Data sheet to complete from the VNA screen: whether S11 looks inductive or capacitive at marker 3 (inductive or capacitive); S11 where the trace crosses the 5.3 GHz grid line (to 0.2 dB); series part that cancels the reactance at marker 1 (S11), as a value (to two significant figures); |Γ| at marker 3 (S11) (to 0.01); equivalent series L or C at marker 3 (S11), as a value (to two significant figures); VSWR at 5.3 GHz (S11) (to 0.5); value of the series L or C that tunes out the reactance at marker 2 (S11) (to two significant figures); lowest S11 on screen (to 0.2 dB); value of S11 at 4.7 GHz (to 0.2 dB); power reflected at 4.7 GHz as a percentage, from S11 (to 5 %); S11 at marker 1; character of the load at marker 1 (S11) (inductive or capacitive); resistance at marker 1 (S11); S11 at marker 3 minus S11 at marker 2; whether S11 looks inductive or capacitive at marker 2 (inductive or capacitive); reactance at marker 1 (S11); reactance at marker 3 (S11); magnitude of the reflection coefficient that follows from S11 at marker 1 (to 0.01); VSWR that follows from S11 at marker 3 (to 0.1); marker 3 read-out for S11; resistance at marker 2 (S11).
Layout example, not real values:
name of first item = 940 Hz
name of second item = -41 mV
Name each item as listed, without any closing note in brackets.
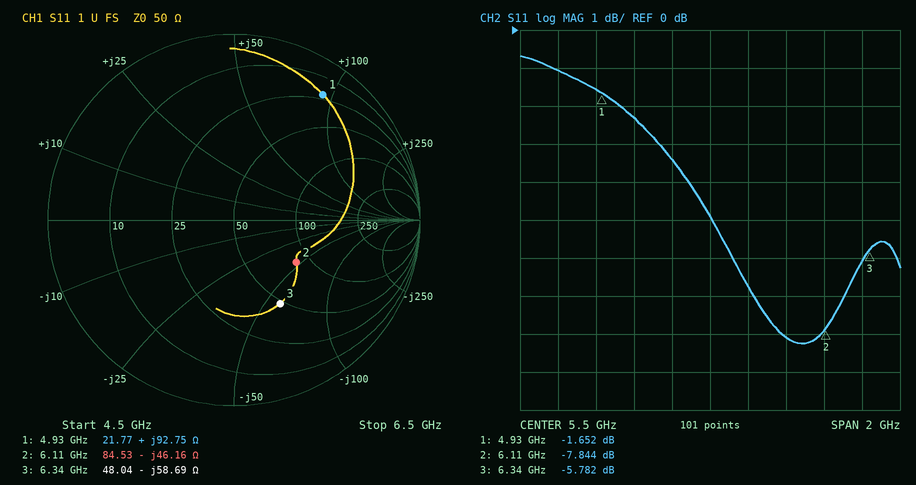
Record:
whether S11 looks inductive or capacitive at marker 3 = capacitive
S11 where the trace crosses the 5.3 GHz grid line = -3.4 dB
series part that cancels the reactance at marker 1 (S11), as a value = 350 fF
|Γ| at marker 3 (S11) = 0.51
equivalent series L or C at marker 3 (S11), as a value = 430 fF
VSWR at 5.3 GHz (S11) = 5.0
value of the series L or C that tunes out the reactance at marker 2 (S11) = 1.2 nH
lowest S11 on screen = -8.2 dB
value of S11 at 4.7 GHz = -1.0 dB
power reflected at 4.7 GHz as a percentage, from S11 = 80 %
S11 at marker 1 = -1.652 dB
character of the load at marker 1 (S11) = inductive
resistance at marker 1 = 21.77 Ω
S11 at marker 3 minus S11 at marker 2 = 2.062 dB
whether S11 looks inductive or capacitive at marker 2 = capacitive
reactance at marker 1 = +92.75 Ω
reactance at marker 3 = -58.69 Ω
magnitude of the reflection coefficient that follows from S11 at marker 1 = 0.83
VSWR that follows from S11 at marker 3 = 3.1
marker 3 read-out for S11 = -5.782 dB
resistance at marker 2 = 84.53 Ω
